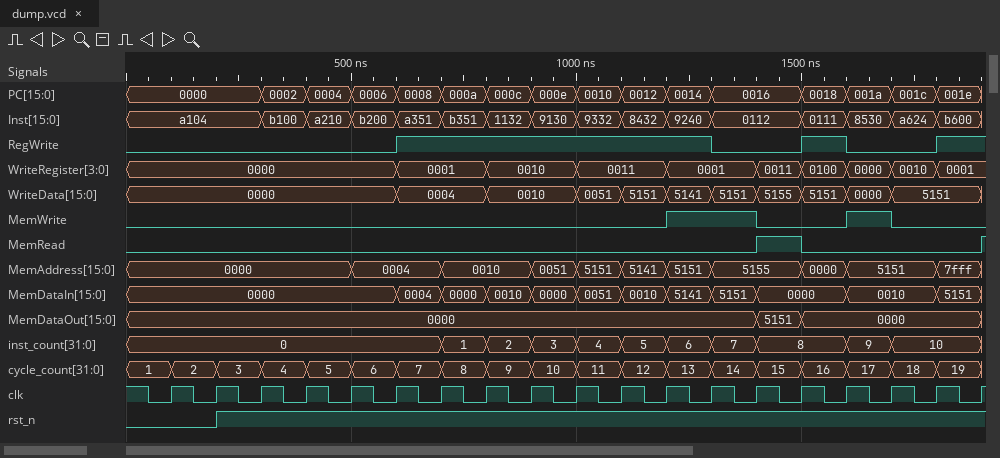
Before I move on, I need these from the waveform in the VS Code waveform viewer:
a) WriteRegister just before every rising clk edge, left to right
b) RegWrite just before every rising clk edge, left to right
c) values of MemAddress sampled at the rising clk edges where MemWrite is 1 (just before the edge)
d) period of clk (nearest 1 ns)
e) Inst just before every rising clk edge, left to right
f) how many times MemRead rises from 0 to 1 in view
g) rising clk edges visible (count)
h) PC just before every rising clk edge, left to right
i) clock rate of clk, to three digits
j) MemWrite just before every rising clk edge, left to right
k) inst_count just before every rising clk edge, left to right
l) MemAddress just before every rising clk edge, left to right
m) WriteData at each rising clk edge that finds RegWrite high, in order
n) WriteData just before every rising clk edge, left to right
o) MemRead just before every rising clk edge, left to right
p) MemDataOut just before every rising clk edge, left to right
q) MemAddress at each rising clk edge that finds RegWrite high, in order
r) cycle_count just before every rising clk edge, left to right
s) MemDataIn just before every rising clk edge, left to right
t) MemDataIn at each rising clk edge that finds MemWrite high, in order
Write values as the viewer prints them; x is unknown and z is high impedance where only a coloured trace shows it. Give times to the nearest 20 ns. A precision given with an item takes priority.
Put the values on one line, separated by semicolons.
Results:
0000, 0000, 0000, 0000, 0000, 0000, 0001, 0001, 0010, 0010, 0011, 0011, 0001, 0001, 0011, 0100, 0000, 0010, 0001; 0 0 0 0 0 0 1 1 1 1 1 1 1 0 0 1 0 0 1; 5151, 5155, 5151; 100 ns; a104, a104, a104, b100, a210, b200, a351, b351, 1132, 9130, 9332, 8432, 9240, 0112, 0112, 0111, 8530, a624, b600; 2; 19; 0000, 0000, 0000, 0002, 0004, 0006, 0008, 000a, 000c, 000e, 0010, 0012, 0014, 0016, 0016, 0018, 001a, 001c, 001e; 10.0 MHz; 0 0 0 0 0 0 0 0 0 0 0 0 1 1 0 0 1 0 0; 0, 0, 0, 0, 0, 0, 0, 1, 2, 3, 4, 5, 6, 7, 8, 8, 9, 10, 10; 0000, 0000, 0000, 0000, 0000, 0004, 0004, 0010, 0010, 0051, 5151, 5141, 5151, 5155, 5155, 0000, 5151, 5151, 7fff; 0004, 0004, 0010, 0010, 0051, 5151, 5141, 5151, 5151; 0000, 0000, 0000, 0000, 0000, 0000, 0004, 0004, 0010, 0010, 0051, 5151, 5141, 5151, 5155, 5151, 0000, 5151, 5151; 0 0 0 0 0 0 0 0 0 0 0 0 0 0 1 0 0 0 0; 0000, 0000, 0000, 0000, 0000, 0000, 0000, 0000, 0000, 0000, 0000, 0000, 0000, 0000, 5151, 0000, 0000, 0000, 0000; 0004, 0010, 0010, 0051, 5151, 5141, 5151, 0000, 7fff; 1, 2, 3, 4, 5, 6, 7, 8, 9, 10, 11, 12, 13, 14, 15, 16, 17, 18, 19; 0000, 0000, 0000, 0000, 0000, 0000, 0004, 0000, 0010, 0000, 0051, 0010, 5141, 5151, 0000, 0000, 0010, 0010, 5151; 5141, 5151, 0010
